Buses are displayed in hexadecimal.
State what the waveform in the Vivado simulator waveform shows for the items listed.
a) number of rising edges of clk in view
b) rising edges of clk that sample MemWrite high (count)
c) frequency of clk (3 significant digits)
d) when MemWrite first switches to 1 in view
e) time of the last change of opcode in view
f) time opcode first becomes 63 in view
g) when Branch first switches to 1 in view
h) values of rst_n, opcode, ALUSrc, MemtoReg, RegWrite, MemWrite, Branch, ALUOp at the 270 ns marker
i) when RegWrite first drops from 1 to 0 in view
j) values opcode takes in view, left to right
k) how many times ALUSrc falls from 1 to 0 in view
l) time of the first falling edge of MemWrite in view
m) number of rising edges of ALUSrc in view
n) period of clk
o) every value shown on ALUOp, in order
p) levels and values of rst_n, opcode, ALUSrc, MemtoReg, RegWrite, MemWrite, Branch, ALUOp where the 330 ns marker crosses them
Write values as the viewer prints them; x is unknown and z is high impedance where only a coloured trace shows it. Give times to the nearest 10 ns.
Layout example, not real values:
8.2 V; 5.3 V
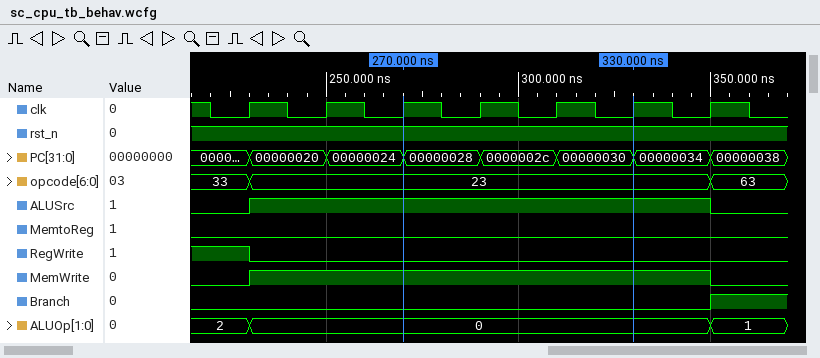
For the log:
7; 6; 50.0 MHz; 230 ns; 350 ns; 350 ns; 350 ns; rst_n=1, opcode=23, ALUSrc=1, MemtoReg=0, RegWrite=0, MemWrite=1, Branch=0, ALUOp=0; 230 ns; 33, 23, 63; 1; 350 ns; 1; 20 ns; 2, 0, 1; rst_n=1, opcode=23, ALUSrc=1, MemtoReg=0, RegWrite=0, MemWrite=1, Branch=0, ALUOp=0
